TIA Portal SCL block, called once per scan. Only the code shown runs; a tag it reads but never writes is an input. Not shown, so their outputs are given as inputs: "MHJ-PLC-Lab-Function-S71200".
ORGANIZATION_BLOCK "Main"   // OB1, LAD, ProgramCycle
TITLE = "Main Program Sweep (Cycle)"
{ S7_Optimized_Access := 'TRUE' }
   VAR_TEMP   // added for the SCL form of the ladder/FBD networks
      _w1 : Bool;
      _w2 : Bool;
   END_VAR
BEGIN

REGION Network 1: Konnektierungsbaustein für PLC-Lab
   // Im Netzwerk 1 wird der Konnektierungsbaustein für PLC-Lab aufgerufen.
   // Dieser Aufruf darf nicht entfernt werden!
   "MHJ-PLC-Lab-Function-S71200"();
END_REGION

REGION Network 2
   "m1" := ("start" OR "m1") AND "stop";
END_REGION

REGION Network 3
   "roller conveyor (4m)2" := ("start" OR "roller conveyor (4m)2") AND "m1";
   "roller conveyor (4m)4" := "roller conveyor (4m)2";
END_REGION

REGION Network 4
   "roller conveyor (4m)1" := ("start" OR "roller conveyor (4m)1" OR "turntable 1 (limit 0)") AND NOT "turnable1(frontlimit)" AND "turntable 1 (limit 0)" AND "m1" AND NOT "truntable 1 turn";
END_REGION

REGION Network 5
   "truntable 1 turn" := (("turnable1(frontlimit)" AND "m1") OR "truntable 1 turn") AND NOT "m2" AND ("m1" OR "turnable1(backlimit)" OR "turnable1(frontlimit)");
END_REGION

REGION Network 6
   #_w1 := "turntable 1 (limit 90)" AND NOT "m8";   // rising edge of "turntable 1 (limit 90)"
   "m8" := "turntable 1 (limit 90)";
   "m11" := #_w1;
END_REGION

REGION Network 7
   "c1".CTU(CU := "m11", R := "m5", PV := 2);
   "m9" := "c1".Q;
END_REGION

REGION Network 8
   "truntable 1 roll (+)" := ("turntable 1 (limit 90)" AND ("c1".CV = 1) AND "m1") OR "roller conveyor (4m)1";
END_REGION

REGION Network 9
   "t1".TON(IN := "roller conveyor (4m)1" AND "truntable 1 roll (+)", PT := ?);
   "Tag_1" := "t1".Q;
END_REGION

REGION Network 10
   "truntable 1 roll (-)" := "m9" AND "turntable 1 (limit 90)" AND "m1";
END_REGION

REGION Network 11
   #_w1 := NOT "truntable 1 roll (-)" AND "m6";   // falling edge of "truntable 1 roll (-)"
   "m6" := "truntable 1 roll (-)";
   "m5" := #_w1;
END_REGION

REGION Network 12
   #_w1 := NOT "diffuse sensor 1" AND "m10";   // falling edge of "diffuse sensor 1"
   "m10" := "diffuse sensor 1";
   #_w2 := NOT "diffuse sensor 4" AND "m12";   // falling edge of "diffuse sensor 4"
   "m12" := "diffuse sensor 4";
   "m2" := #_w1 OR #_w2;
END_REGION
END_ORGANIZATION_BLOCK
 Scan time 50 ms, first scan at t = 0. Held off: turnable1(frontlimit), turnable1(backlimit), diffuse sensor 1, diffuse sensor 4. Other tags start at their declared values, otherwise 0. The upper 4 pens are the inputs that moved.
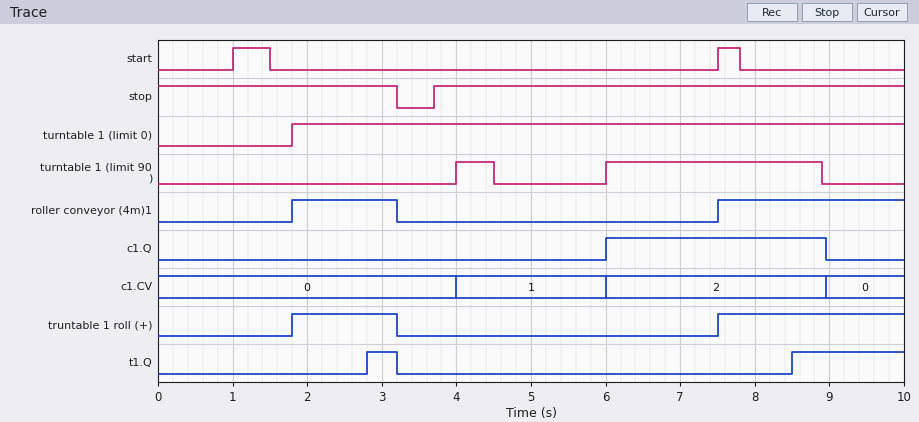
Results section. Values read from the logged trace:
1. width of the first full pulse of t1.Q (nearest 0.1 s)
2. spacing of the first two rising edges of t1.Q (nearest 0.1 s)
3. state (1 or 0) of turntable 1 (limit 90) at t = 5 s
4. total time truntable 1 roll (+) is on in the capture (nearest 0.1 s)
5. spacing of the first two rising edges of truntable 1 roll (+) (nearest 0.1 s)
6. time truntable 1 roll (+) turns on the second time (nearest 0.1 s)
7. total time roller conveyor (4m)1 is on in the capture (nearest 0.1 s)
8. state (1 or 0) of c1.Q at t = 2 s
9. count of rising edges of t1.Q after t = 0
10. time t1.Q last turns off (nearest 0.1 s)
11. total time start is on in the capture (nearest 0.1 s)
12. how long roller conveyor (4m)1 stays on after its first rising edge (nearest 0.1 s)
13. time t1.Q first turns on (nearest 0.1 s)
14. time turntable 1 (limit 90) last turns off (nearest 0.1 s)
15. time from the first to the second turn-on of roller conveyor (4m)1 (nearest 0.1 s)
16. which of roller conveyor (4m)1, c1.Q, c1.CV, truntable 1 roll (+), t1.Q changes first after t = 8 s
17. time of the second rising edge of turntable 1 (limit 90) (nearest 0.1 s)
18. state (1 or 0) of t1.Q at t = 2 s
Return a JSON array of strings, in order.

["0.4 s", "5.7 s", "0", "3.9 s", "5.7 s", "7.5 s", "3.9 s", "0", "2", "3.2 s", "0.8 s", "1.4 s", "2.8 s", "8.9 s", "5.7 s", "t1.Q", "6.0 s", "0"]
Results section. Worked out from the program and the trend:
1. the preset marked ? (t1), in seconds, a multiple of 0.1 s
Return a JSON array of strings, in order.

["1.0 s"]
